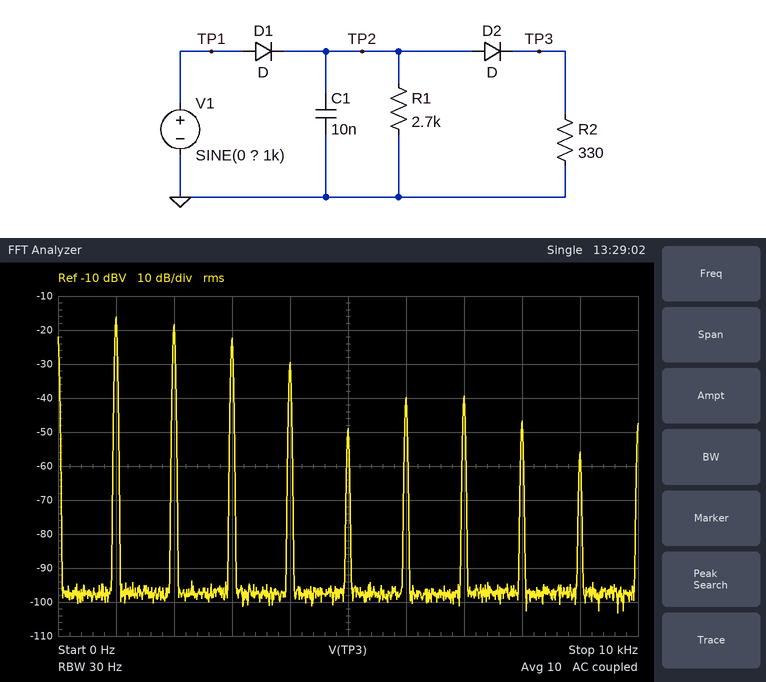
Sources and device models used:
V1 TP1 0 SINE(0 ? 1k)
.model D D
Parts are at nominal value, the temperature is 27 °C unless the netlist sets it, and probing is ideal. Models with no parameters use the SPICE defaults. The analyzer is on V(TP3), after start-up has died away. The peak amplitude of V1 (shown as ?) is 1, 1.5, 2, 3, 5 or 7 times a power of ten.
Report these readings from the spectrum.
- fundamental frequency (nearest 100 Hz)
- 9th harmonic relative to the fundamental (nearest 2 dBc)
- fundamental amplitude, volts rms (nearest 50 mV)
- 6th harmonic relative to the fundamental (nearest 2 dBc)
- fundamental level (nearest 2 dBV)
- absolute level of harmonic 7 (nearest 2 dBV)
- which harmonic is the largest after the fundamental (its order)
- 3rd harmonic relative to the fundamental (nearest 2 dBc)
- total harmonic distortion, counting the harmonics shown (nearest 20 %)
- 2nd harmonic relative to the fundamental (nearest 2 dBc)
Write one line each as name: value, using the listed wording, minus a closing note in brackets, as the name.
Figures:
fundamental frequency: 1.0 kHz
9th harmonic relative to the fundamental: -40 dBc
fundamental amplitude, volts rms: 150 mV
6th harmonic relative to the fundamental: -24 dBc
fundamental level: -16 dBV
absolute level of harmonic 7: -40 dBV
which harmonic is the largest after the fundamental: 2
3rd harmonic relative to the fundamental: -6 dBc
total harmonic distortion, counting the harmonics shown: 100 %
2nd harmonic relative to the fundamental: -2 dBc
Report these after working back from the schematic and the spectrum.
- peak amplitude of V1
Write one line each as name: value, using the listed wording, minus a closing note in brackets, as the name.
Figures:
peak amplitude of V1: 2 V
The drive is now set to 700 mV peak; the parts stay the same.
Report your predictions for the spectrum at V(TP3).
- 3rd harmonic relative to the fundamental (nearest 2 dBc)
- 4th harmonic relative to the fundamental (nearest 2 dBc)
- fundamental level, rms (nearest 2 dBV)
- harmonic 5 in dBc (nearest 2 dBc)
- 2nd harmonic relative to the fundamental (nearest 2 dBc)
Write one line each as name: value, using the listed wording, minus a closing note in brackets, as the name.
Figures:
3rd harmonic relative to the fundamental: 0 dBc
4th harmonic relative to the fundamental: 0 dBc
fundamental level, rms: -180 dBV
harmonic 5 in dBc: 0 dBc
2nd harmonic relative to the fundamental: 0 dBc
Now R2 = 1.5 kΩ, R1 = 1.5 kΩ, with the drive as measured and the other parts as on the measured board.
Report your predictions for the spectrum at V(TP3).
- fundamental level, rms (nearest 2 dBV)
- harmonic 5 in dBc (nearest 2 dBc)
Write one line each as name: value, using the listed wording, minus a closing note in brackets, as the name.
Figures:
fundamental level, rms: -16 dBV
harmonic 5 in dBc: -50 dBc
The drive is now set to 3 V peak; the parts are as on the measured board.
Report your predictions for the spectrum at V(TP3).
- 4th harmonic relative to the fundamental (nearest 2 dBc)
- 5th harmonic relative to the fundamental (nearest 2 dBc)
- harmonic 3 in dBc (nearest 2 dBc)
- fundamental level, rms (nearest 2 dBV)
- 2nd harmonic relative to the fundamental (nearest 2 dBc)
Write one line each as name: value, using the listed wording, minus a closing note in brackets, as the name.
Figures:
4th harmonic relative to the fundamental: -34 dBc
5th harmonic relative to the fundamental: -22 dBc
harmonic 3 in dBc: -10 dBc
fundamental level, rms: -6 dBV
2nd harmonic relative to the fundamental: -4 dBc
